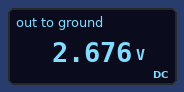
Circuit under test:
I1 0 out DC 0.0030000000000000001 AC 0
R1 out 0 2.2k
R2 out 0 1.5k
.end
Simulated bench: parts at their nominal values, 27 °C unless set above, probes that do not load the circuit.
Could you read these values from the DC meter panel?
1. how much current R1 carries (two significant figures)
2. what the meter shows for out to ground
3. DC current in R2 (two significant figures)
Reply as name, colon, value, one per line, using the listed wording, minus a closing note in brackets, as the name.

how much current R1 carries: 1.2 mA
what the meter shows for out to ground: 2.676 V
DC current in R2: 1.8 mA
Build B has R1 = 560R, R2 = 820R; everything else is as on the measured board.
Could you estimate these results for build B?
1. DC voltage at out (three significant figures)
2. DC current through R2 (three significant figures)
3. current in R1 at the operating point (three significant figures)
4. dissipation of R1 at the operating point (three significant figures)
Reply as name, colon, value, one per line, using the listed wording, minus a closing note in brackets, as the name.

DC voltage at out: 998 mV
DC current through R2: 1.22 mA
current in R1 at the operating point: 1.78 mA
dissipation of R1 at the operating point: 1.78 mW
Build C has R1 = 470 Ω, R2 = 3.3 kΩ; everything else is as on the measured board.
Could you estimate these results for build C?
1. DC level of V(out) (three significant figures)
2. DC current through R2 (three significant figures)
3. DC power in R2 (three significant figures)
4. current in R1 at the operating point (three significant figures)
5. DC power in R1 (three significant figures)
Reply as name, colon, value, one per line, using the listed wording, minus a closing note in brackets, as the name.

DC level of V(out): 1.23 V
DC current through R2: 374 µA
DC power in R2: 462 µW
current in R1 at the operating point: 2.63 mA
DC power in R1: 3.24 mW
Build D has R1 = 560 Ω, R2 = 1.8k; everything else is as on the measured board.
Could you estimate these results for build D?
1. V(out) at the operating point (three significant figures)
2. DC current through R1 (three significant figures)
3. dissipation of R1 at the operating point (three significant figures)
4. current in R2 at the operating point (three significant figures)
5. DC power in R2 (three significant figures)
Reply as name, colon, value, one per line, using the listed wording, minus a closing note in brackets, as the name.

V(out) at the operating point: 1.28 V
DC current through R1: 2.29 mA
dissipation of R1 at the operating point: 2.93 mW
current in R2 at the operating point: 712 µA
DC power in R2: 912 µW
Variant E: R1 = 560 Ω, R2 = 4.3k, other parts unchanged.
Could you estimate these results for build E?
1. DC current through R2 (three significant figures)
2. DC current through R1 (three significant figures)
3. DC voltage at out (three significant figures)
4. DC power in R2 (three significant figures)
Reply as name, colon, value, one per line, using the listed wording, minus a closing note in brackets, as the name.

DC current through R2: 346 µA
DC current through R1: 2.65 mA
DC voltage at out: 1.49 V
DC power in R2: 514 µW
